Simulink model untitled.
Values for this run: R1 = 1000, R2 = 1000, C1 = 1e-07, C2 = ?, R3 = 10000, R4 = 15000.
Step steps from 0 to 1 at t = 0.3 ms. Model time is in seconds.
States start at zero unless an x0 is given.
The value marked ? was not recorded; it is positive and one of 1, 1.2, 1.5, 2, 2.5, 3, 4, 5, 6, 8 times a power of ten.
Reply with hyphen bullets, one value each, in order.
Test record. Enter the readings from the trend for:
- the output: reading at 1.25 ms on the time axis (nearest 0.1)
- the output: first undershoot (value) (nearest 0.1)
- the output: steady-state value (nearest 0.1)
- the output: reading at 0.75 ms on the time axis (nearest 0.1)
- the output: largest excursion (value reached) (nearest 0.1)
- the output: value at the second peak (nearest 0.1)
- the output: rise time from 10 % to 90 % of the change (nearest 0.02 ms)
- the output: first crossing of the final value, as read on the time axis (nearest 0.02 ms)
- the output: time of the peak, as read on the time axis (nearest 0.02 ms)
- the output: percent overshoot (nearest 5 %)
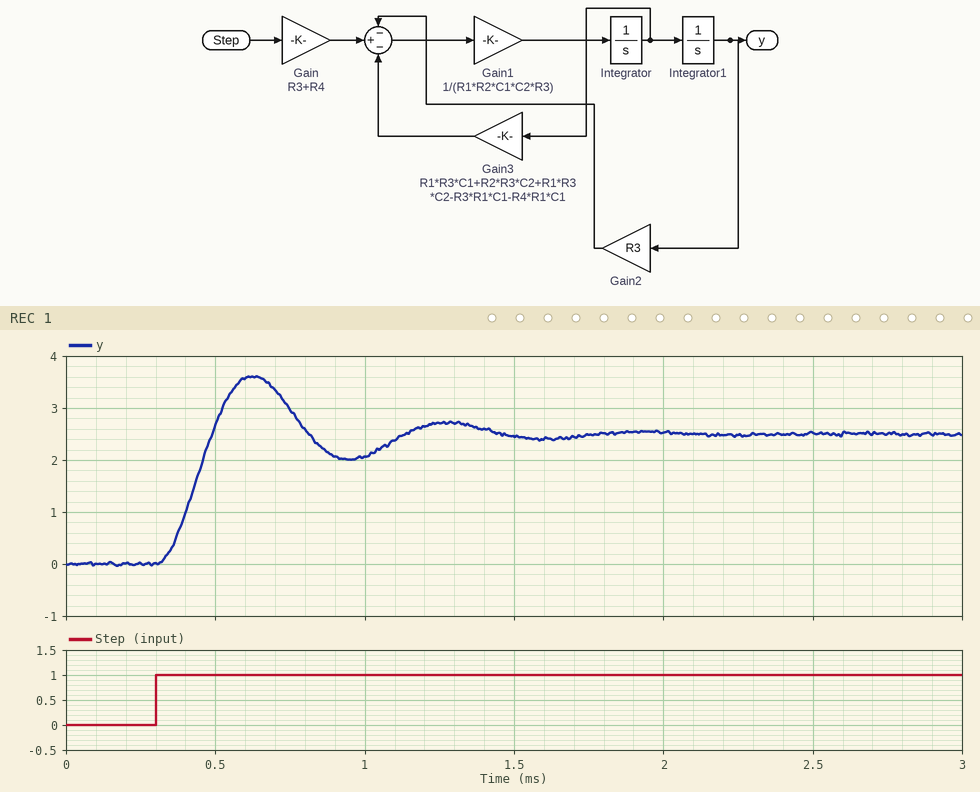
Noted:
- 2.7
- 2.0
- 2.5
- 3.0
- 3.6
- 2.7
- 0.12 ms
- 0.48 ms
- 0.62 ms
- 45 %
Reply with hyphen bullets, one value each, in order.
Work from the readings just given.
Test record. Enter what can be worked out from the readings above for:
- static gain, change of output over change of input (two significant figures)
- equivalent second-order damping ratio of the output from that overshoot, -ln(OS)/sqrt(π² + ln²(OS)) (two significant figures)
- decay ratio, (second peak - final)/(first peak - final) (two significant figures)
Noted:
- 2.5
- 0.25
- 0.18
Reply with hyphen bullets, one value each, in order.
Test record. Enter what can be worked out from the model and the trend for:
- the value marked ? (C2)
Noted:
- 1e-07
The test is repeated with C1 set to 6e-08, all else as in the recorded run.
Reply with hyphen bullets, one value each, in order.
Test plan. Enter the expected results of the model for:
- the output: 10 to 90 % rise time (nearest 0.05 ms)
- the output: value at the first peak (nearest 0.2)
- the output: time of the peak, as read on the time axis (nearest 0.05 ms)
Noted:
- 0.15 ms
- 2.6
- 0.65 ms
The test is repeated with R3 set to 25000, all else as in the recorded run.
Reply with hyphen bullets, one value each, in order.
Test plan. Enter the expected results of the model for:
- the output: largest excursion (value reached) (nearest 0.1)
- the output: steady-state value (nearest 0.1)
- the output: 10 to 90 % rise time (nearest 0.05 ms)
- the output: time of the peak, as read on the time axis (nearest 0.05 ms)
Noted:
- 1.7
- 1.6
- 0.20 ms
- 0.75 ms
